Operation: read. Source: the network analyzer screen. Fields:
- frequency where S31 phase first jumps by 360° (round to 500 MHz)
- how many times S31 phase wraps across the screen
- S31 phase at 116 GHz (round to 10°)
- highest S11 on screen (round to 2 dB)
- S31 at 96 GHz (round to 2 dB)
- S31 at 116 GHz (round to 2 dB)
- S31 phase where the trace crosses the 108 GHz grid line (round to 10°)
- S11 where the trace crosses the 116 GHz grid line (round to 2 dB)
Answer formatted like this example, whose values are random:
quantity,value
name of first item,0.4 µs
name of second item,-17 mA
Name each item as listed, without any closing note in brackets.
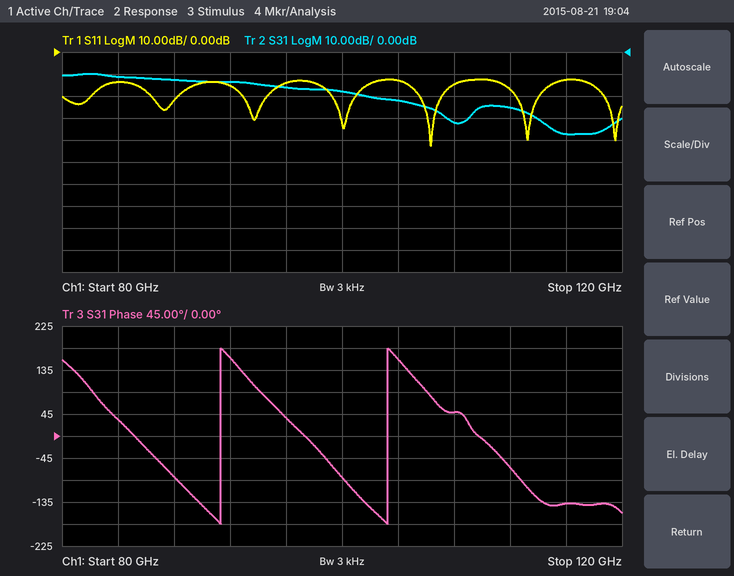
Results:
quantity,value
frequency where S31 phase first jumps by 360°,91.5 GHz
how many times S31 phase wraps across the screen,2
S31 phase at 116 GHz,-140°
highest S11 on screen,-12 dB
S31 at 96 GHz,-16 dB
S31 at 116 GHz,-38 dB
S31 phase where the trace crosses the 108 GHz grid line,50°
S11 where the trace crosses the 116 GHz grid line,-12 dB
